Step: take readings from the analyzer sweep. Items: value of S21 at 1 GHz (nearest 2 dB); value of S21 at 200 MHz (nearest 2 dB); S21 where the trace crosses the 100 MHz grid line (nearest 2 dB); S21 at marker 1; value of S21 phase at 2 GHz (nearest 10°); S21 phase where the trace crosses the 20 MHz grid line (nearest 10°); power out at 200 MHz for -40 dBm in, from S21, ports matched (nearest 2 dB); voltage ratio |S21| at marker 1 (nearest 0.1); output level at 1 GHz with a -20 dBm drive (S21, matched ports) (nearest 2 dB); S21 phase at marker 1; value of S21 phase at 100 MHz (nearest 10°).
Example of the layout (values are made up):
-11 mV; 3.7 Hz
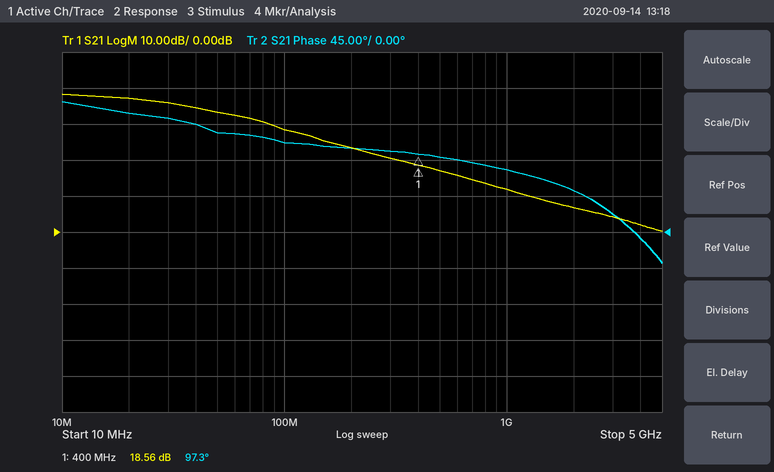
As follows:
12 dB; 24 dB; 28 dB; 18.56 dB; 50°; 150°; -16 dBm; 8.5; -8 dBm; 97.3°; 110°
